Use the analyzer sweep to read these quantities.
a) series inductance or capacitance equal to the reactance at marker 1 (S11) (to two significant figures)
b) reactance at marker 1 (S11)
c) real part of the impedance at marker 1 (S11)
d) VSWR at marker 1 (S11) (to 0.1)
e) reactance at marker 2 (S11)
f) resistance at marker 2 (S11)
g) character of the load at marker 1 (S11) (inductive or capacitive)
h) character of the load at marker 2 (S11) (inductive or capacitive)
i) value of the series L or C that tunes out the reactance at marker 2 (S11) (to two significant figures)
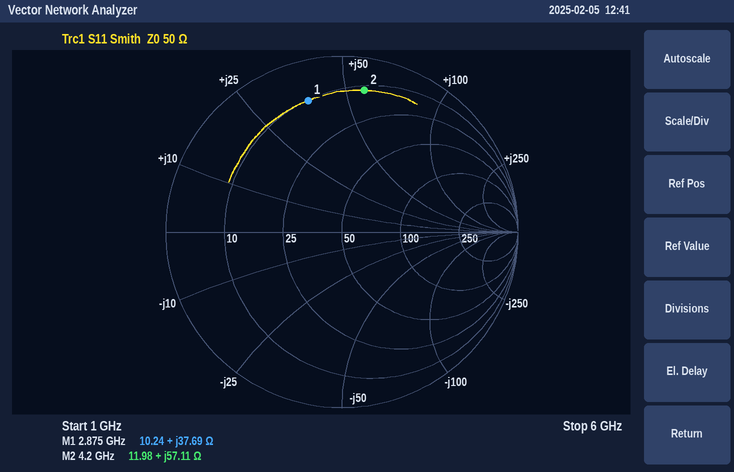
2.1 nH
+37.69 Ω
10.24 Ω
7.7
+57.11 Ω
11.98 Ω
inductive
inductive
660 fF
